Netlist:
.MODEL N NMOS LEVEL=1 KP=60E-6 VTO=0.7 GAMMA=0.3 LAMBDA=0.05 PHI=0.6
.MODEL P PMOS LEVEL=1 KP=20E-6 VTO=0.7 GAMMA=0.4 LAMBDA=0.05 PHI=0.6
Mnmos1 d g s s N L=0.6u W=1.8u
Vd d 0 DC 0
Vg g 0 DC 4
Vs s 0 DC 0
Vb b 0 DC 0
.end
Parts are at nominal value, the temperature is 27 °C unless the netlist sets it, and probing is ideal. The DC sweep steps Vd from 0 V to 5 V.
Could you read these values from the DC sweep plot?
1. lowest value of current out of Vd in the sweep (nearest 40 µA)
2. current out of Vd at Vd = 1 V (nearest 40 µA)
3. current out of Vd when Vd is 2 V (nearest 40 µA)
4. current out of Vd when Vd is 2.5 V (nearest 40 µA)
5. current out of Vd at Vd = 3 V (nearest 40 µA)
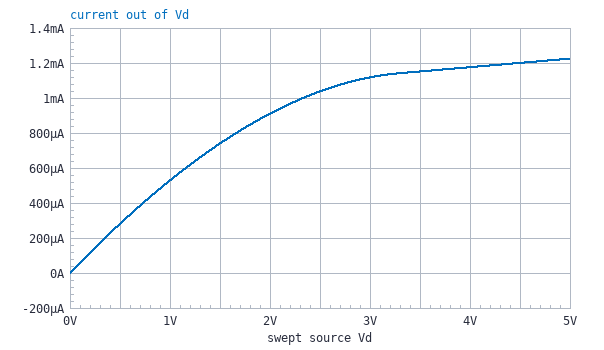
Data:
0 A
520 µA
920 µA
1.04 mA
1.12 mA
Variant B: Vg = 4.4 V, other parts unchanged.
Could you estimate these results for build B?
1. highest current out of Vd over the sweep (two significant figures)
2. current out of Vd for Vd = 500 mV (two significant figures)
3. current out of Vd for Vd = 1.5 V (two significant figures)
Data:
1.5 mA
320 µA
860 µA
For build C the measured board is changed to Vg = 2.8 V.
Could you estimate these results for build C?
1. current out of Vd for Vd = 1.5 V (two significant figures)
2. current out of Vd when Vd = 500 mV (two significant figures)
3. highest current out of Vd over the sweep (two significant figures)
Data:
390 µA
170 µA
500 µA
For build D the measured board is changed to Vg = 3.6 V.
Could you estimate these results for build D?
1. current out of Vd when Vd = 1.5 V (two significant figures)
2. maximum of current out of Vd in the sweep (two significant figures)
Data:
620 µA
950 µA
